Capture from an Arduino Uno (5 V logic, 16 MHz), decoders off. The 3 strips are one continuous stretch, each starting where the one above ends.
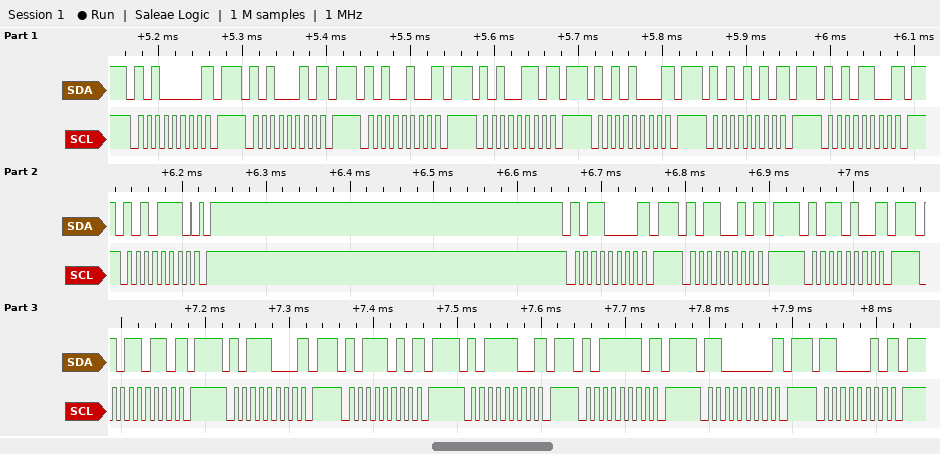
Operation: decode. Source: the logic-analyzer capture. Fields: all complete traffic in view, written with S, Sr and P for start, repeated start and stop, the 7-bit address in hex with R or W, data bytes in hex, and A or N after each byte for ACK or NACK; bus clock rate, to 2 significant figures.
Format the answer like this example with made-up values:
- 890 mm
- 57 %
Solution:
- S 50W N P S 51W N P S 52W N P S 53W N P S 54W N P S 55W N P S 56W N P S 57W A P S 58W N P S 59W N P S 5AW N P S 5BW N P S 5CW N P S 5DW N P S 5EW N P S 5FW N P S 60W N P S 61W N P
- 100 kHz
